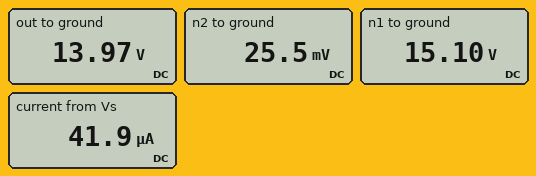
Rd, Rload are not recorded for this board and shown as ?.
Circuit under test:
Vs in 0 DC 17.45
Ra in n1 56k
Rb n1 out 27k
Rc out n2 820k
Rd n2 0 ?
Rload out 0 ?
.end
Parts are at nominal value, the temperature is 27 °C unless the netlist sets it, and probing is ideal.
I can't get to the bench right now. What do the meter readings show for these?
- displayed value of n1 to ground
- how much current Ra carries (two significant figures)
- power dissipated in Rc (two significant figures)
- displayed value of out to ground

15.10 V
42 µA
240 µW
13.97 V
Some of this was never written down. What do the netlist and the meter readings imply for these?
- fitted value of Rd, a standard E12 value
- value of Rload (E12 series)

1.5 kΩ
560 kΩ
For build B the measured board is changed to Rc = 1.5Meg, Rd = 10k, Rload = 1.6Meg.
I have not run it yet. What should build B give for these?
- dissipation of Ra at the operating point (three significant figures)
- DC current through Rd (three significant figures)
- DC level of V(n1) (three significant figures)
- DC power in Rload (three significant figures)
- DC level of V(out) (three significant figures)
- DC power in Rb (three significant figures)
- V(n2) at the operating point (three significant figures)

23.1 µW
10.4 µA
16.3 V
155 µW
15.8 V
11.1 µW
104 mV
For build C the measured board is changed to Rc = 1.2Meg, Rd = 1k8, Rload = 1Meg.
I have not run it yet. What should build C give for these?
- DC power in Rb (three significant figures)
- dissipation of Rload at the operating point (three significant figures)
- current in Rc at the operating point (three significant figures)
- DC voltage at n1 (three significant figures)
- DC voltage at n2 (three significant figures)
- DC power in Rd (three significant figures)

20.8 µW
229 µW
12.6 µA
15.9 V
22.7 mV
286 nW
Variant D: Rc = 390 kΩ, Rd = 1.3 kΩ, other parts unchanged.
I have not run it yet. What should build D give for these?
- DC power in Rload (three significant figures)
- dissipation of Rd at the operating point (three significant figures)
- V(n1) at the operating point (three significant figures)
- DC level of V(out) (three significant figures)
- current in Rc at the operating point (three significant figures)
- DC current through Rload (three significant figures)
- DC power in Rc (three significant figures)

294 µW
1.40 µW
14.3 V
12.8 V
32.8 µA
22.9 µA
419 µW
